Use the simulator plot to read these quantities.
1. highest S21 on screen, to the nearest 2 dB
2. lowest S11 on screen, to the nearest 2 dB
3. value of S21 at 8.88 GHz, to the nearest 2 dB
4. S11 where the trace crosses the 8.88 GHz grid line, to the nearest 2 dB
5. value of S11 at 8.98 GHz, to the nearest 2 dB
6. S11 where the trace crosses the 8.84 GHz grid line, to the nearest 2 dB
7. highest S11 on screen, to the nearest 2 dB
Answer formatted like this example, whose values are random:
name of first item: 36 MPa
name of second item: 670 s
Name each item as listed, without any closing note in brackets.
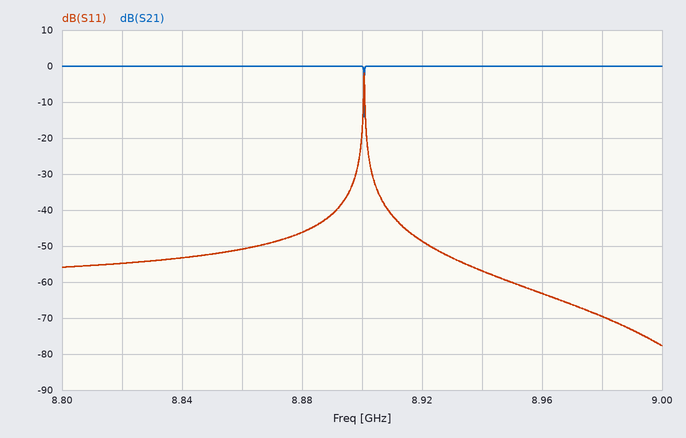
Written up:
highest S21 on screen, to the nearest 2 dB: 0 dB
lowest S11 on screen, to the nearest 2 dB: -78 dB
value of S21 at 8.88 GHz, to the nearest 2 dB: 0 dB
S11 where the trace crosses the 8.88 GHz grid line, to the nearest 2 dB: -46 dB
value of S11 at 8.98 GHz, to the nearest 2 dB: -70 dB
S11 where the trace crosses the 8.84 GHz grid line, to the nearest 2 dB: -54 dB
highest S11 on screen, to the nearest 2 dB: -2 dB
